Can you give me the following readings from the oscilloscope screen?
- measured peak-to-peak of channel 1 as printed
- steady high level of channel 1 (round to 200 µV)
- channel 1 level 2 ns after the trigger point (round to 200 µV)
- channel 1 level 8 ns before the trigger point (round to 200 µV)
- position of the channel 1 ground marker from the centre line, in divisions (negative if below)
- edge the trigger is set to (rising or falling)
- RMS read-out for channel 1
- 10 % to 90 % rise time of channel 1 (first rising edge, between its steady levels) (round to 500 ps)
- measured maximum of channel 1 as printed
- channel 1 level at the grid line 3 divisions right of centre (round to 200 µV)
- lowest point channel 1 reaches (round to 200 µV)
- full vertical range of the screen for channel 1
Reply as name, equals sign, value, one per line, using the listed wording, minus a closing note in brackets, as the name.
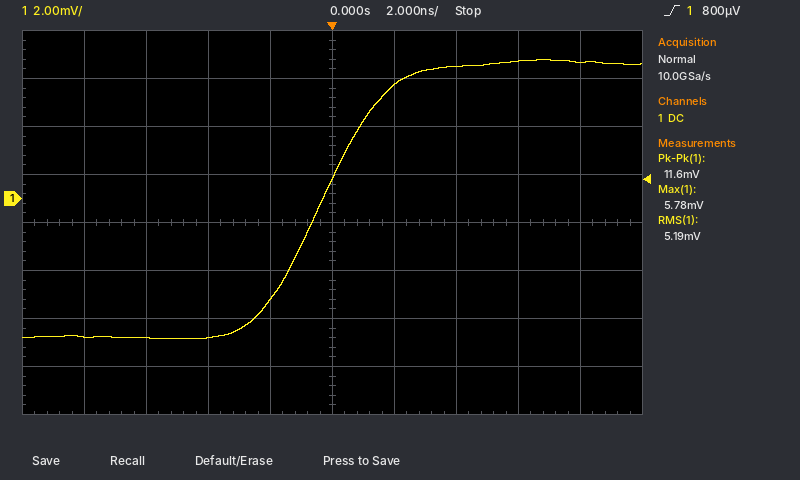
measured peak-to-peak of channel 1 as printed = 11.6 mV
steady high level of channel 1 = 5.6 mV
channel 1 level 2 ns after the trigger point = 4.8 mV
channel 1 level 8 ns before the trigger point = -5.8 mV
position of the channel 1 ground marker from the centre line, in divisions = +0.5 div
edge the trigger is set to = rising
RMS read-out for channel 1 = 5.19 mV
10 % to 90 % rise time of channel 1 (first rising edge, between its steady levels) = 4.0 ns
measured maximum of channel 1 as printed = 5.78 mV
channel 1 level at the grid line 3 divisions right of centre = 5.8 mV
lowest point channel 1 reaches = -5.8 mV
full vertical range of the screen for channel 1 = 16 mV
